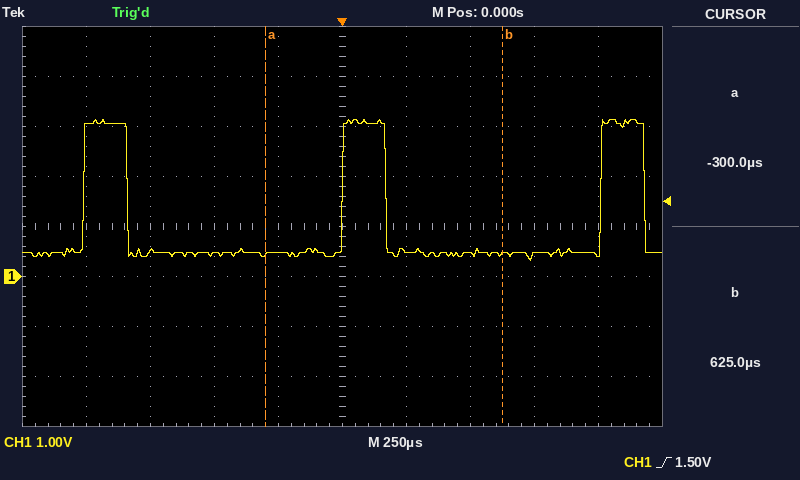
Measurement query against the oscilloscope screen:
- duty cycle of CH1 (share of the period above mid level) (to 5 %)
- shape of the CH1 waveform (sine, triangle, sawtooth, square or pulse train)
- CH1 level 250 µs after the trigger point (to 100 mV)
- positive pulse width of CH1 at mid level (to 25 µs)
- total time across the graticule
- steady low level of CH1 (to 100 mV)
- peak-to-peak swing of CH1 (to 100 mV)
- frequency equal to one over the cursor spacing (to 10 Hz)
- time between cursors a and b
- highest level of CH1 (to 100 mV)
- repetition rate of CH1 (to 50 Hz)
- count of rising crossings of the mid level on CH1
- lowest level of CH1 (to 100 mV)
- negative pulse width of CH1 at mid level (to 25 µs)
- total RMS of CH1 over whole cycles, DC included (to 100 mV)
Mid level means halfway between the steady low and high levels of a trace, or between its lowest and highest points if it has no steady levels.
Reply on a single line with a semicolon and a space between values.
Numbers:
15 %; pulse train; 500 mV; 175 µs; 2.5 ms; 500 mV; 2.8 V; 1.08 kHz; 925 µs; 3.1 V; 1.00 kHz; 3; 300 mV; 850 µs; 1.3 V
